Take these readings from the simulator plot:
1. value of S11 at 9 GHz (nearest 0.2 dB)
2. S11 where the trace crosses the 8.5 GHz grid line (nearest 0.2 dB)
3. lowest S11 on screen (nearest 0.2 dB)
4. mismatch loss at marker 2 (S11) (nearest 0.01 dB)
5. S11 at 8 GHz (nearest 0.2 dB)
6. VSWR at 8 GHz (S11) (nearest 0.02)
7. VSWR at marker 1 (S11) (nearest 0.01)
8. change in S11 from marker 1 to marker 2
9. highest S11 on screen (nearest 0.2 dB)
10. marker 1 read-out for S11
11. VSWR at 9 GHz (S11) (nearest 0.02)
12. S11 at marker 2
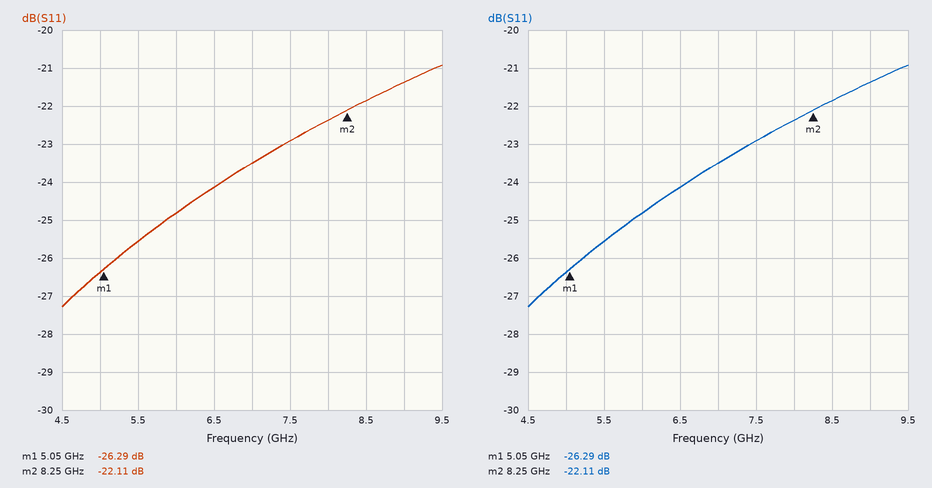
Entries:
-21.4 dB
-21.8 dB
-27.2 dB
0.03 dB
-22.4 dB
1.16
1.10
4.18 dB
-21.0 dB
-26.29 dB
1.18
-22.11 dB
